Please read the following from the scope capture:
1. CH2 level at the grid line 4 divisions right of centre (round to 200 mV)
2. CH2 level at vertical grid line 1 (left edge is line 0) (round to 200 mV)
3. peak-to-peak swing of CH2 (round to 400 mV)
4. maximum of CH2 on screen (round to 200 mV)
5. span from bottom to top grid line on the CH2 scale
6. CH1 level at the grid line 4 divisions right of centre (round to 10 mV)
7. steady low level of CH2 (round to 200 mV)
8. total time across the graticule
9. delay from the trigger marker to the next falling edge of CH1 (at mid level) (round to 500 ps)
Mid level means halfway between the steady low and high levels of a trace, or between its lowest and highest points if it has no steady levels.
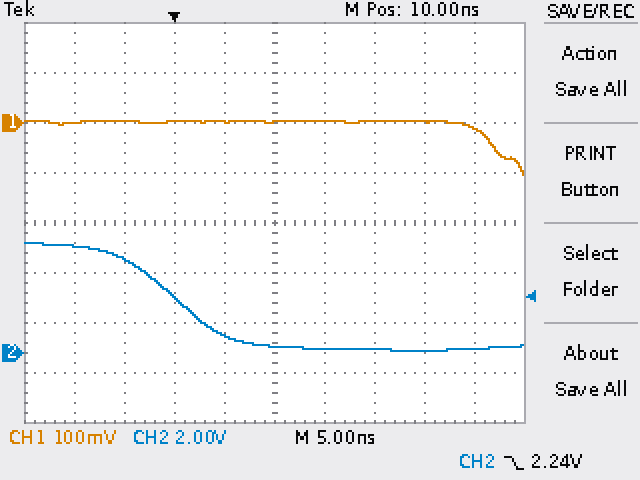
200 mV
4.2 V
4.4 V
4.4 V
16 V
-10 mV
200 mV
50 ns
32.0 ns
